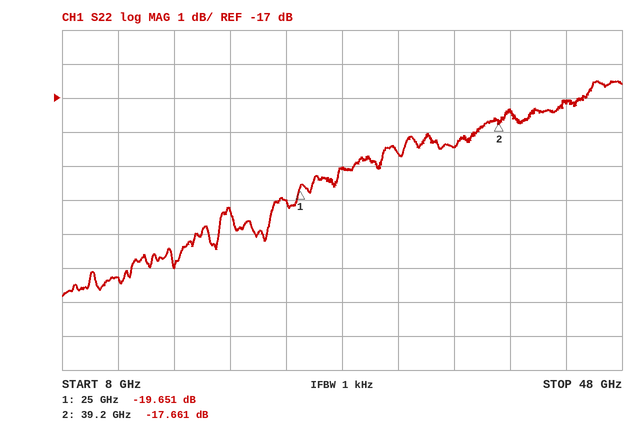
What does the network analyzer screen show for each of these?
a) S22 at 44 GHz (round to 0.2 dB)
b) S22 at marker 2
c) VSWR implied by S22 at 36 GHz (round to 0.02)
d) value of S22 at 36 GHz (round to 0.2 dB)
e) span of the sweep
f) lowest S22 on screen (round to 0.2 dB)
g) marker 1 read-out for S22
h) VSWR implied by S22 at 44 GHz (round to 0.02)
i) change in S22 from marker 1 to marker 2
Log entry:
-17.2 dB
-17.661 dB
1.28
-18.4 dB
40 GHz
-22.8 dB
-19.651 dB
1.32
1.990 dB
